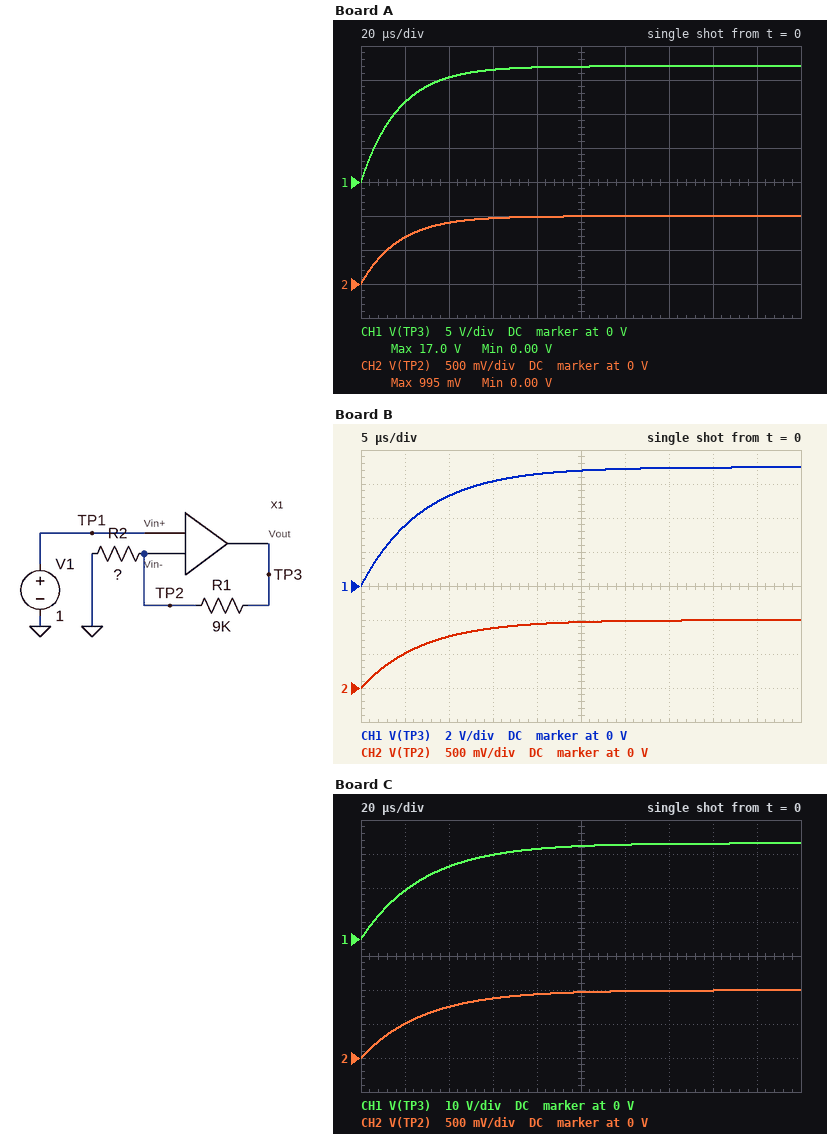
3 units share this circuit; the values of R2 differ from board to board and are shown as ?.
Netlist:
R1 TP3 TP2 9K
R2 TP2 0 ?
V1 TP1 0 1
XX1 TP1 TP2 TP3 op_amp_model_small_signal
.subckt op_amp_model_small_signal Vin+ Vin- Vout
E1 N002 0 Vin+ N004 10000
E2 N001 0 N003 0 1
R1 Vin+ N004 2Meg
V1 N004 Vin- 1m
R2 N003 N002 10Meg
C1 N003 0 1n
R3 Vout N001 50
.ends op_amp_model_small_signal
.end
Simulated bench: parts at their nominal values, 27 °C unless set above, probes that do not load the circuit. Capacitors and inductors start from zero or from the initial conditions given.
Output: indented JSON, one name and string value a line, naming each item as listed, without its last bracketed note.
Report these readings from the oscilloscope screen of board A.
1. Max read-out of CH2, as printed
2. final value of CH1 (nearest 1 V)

{
  "Max read-out of CH2, as printed": "995 mV",
  "final value of CH1": "17 V"
}
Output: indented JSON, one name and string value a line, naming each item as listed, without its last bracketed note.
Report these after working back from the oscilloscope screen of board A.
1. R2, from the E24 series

{
  "R2, from the E24 series": "560 Ω"
}
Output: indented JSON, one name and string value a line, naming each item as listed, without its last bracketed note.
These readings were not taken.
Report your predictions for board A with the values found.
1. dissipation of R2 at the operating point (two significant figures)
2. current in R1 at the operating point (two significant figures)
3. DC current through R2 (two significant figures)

{
  "dissipation of R2 at the operating point": "1.8 mW",
  "current in R1 at the operating point": "1.8 mA",
  "DC current through R2": "1.8 mA"
}
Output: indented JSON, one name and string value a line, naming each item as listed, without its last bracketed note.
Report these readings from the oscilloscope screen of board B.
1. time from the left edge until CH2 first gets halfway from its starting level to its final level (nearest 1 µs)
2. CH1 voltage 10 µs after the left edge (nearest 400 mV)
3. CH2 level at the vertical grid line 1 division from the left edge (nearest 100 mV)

{
  "time from the left edge until CH2 first gets halfway from its starting level to its final level": "5 µs",
  "CH1 voltage 10 µs after the left edge": "5.2 V",
  "CH2 level at the vertical grid line 1 division from the left edge": "500 mV"
}
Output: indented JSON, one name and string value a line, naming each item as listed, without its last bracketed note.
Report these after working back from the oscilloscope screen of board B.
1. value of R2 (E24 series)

{
  "value of R2": "1.5 kΩ"
}
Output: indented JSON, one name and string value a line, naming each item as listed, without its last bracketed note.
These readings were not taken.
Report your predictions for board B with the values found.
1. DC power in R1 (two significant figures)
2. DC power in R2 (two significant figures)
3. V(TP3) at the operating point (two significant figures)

{
  "DC power in R1": "4.0 mW",
  "DC power in R2": "660 µW",
  "V(TP3) at the operating point": "7.0 V"
}
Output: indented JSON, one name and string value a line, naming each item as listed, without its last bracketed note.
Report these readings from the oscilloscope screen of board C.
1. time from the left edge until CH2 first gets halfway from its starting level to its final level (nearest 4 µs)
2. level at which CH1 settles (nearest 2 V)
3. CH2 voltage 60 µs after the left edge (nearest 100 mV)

{
  "time from the left edge until CH2 first gets halfway from its starting level to its final level": "20 µs",
  "level at which CH1 settles": "28 V",
  "CH2 voltage 60 µs after the left edge": "900 mV"
}
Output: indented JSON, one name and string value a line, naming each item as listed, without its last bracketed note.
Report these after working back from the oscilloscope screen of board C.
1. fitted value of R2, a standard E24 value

{
  "fitted value of R2, a standard E24 value": "330 Ω"
}
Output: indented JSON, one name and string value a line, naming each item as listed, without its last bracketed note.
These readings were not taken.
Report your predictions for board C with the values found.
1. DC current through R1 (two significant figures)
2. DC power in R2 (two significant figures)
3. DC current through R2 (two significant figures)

{
  "DC current through R1": "3.0 mA",
  "DC power in R2": "3.0 mW",
  "DC current through R2": "3.0 mA"
}
